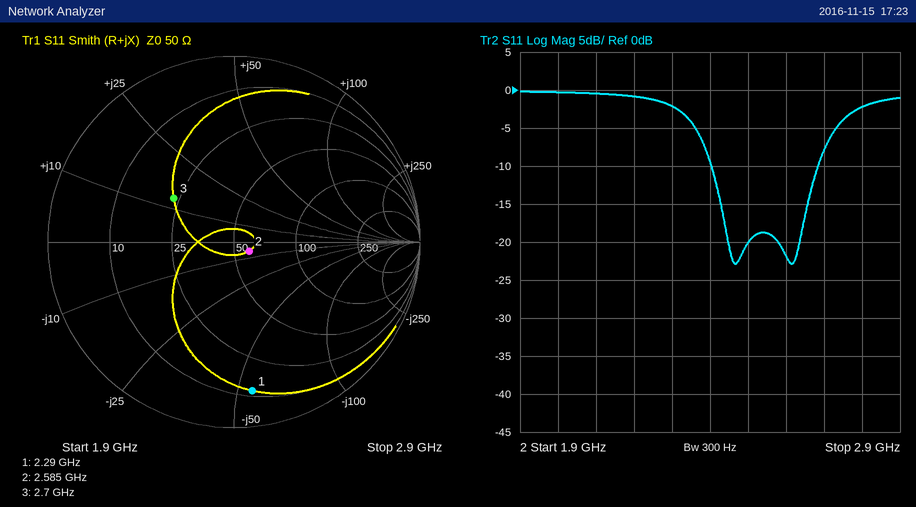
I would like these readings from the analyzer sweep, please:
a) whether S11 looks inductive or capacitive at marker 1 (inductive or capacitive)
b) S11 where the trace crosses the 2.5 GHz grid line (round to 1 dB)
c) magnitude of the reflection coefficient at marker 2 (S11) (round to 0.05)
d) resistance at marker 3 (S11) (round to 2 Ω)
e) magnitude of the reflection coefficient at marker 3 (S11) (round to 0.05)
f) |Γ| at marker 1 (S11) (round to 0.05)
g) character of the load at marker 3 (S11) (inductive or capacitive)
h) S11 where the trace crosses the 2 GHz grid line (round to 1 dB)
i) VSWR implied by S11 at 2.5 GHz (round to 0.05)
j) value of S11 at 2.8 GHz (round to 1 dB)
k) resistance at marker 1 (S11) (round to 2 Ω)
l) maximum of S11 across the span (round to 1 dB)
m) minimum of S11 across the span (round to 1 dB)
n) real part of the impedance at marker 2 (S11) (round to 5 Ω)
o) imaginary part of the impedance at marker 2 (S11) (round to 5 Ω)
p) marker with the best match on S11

capacitive
-20 dB
0.10
24 Ω
0.40
0.80
inductive
0 dB
1.20
-2 dB
12 Ω
0 dB
-23 dB
60 Ω
-5 Ω
marker 2
